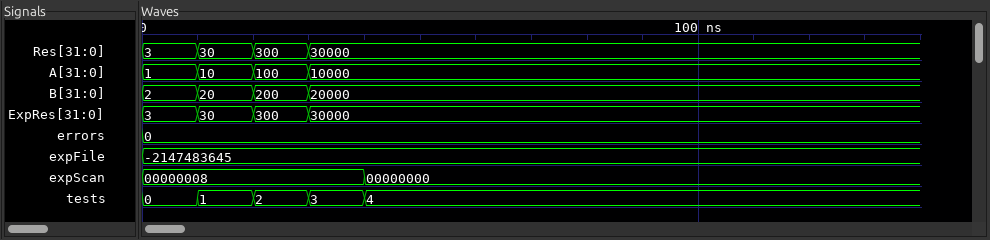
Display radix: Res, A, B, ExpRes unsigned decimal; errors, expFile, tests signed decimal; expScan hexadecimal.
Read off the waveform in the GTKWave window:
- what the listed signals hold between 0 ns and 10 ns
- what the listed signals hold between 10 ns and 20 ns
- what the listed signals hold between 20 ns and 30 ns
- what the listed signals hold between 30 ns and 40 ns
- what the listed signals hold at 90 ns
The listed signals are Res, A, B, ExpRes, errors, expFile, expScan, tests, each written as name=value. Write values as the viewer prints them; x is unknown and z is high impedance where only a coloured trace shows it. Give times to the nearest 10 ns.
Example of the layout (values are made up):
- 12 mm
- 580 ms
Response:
- Res=3, A=1, B=2, ExpRes=3, errors=0, expFile=-2147483645, expScan=00000008, tests=0
- Res=30, A=10, B=20, ExpRes=30, errors=0, expFile=-2147483645, expScan=00000008, tests=1
- Res=300, A=100, B=200, ExpRes=300, errors=0, expFile=-2147483645, expScan=00000008, tests=2
- Res=30000, A=10000, B=20000, ExpRes=30000, errors=0, expFile=-2147483645, expScan=00000008, tests=3
- Res=30000, A=10000, B=20000, ExpRes=30000, errors=0, expFile=-2147483645, expScan=00000000, tests=4
